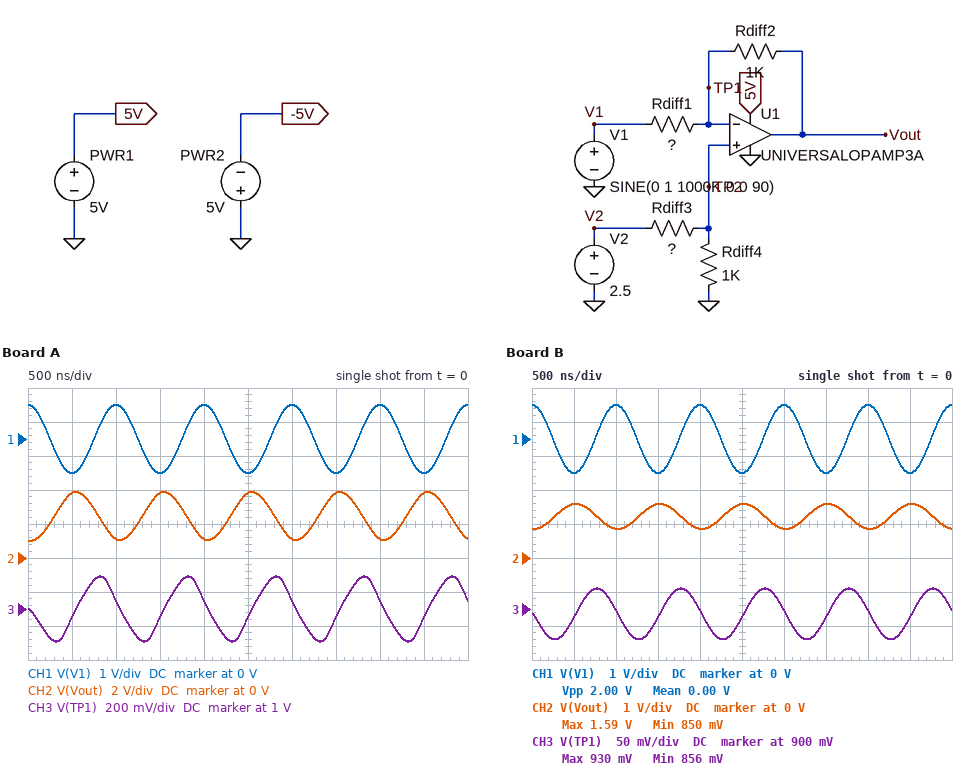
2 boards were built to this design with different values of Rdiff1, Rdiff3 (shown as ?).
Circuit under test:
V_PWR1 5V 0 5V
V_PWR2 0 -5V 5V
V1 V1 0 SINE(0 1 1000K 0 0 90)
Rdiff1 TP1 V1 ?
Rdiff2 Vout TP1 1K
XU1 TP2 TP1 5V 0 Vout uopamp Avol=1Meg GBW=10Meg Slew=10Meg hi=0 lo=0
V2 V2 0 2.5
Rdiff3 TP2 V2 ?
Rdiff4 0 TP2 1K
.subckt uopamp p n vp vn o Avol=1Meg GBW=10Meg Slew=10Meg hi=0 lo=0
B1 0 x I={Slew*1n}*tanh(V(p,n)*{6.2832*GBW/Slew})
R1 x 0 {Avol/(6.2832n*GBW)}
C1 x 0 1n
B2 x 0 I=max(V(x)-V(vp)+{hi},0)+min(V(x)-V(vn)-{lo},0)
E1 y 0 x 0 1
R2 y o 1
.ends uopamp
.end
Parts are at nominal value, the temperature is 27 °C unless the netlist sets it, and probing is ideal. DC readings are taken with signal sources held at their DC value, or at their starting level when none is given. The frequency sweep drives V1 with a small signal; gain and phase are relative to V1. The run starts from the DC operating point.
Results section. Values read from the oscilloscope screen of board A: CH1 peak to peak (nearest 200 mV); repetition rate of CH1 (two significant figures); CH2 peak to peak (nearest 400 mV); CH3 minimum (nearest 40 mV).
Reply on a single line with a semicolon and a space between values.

2.0 V; 1.0 MHz; 2.8 V; 800 mV
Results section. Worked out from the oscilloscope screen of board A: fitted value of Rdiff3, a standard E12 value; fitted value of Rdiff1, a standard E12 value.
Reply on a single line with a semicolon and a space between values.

1.5 kΩ; 680 Ω
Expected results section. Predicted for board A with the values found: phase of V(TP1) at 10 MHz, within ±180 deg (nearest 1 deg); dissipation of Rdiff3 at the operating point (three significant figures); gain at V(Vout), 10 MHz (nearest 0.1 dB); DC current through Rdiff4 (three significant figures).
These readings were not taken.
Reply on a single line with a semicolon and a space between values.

22 deg; 1.50 mW; -5.2 dB; 1.00 mA
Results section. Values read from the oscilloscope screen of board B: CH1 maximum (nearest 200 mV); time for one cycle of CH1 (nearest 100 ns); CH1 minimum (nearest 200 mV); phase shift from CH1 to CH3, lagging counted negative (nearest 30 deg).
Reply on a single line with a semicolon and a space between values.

1.0 V; 1.0 µs; -1.0 V; 90 deg
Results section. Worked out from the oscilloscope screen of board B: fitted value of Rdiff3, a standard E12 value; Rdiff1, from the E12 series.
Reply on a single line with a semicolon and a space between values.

1.8 kΩ; 2.7 kΩ
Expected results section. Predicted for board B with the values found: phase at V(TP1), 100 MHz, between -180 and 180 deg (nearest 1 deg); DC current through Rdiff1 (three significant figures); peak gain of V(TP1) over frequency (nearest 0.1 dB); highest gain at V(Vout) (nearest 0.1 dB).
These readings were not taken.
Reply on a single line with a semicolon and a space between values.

4 deg; 39.7 µA; -11.4 dB; -8.6 dB
